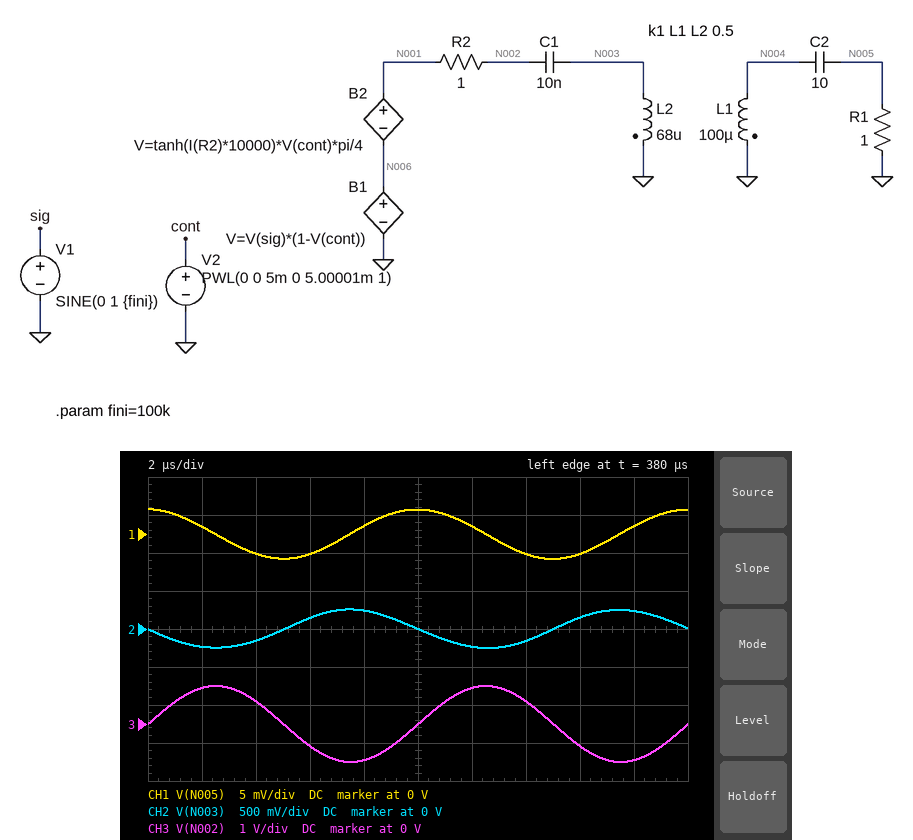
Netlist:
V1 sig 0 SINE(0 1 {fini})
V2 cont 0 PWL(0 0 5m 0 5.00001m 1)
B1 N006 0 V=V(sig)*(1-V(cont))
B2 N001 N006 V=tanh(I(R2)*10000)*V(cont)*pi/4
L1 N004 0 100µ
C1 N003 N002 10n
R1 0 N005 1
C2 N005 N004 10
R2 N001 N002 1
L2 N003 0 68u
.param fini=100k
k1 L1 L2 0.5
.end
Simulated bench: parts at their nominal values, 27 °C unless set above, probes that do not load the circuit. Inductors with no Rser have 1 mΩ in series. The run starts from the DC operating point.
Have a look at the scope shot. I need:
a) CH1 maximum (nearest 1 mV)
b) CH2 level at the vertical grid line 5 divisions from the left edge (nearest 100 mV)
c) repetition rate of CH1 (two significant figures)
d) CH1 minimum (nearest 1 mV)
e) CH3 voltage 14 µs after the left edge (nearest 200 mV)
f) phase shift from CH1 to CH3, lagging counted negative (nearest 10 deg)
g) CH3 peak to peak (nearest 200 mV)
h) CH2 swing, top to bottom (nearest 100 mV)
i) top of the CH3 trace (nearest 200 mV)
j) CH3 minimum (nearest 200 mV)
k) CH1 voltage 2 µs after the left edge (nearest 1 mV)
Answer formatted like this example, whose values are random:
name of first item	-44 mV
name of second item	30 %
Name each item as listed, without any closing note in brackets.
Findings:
CH1 maximum	3 mV
CH2 level at the vertical grid line 5 divisions from the left edge	0 V
repetition rate of CH1	100 kHz
CH1 minimum	-3 mV
CH3 voltage 14 µs after the left edge	600 mV
phase shift from CH1 to CH3, lagging counted negative	-90 deg
CH3 peak to peak	2.0 V
CH2 swing, top to bottom	500 mV
top of the CH3 trace	1.0 V
CH3 minimum	-1.0 V
CH1 voltage 2 µs after the left edge	1 mV
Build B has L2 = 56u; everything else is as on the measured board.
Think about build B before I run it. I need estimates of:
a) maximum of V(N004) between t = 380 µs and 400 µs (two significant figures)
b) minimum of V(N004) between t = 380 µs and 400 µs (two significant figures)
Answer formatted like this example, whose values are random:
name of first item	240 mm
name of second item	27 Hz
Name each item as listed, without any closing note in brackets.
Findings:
maximum of V(N004) between t = 380 µs and 400 µs	2.8 mV
minimum of V(N004) between t = 380 µs and 400 µs	-2.8 mV
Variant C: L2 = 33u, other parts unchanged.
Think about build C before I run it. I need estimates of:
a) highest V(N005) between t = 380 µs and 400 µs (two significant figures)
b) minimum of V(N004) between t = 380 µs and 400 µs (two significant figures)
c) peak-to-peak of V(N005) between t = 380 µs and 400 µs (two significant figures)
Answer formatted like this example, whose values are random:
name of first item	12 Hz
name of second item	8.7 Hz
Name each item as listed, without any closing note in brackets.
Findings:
highest V(N005) between t = 380 µs and 400 µs	2.0 mV
minimum of V(N004) between t = 380 µs and 400 µs	-2.0 mV
peak-to-peak of V(N005) between t = 380 µs and 400 µs	4.0 mV
